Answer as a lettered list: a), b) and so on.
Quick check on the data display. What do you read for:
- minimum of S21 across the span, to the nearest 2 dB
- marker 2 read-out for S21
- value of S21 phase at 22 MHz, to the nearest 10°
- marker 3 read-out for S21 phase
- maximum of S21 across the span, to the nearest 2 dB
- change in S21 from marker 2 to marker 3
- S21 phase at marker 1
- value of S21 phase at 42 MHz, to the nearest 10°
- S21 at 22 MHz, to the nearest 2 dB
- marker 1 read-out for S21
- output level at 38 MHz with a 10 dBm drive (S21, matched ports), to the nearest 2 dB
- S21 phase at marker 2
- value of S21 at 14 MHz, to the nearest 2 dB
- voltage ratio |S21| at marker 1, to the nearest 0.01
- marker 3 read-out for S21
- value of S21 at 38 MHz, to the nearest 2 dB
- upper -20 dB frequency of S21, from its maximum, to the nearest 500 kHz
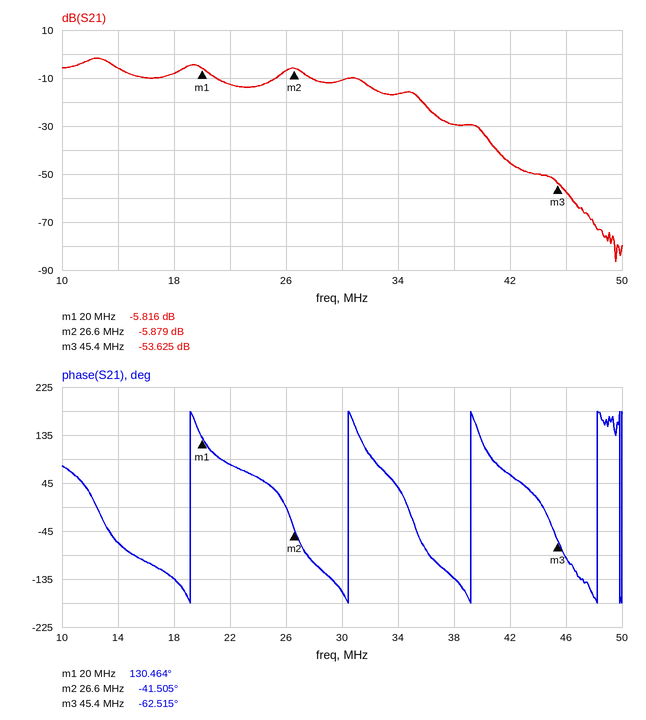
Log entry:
a) -86 dB
b) -5.879 dB
c) 80°
d) -62.515°
e) -2 dB
f) -47.746 dB
g) 130.464°
h) 60°
i) -12 dB
j) -5.816 dB
k) -20 dBm
l) -41.505°
m) -6 dB
n) 0.51
o) -53.625 dB
p) -30 dB
q) 36.0 MHz
